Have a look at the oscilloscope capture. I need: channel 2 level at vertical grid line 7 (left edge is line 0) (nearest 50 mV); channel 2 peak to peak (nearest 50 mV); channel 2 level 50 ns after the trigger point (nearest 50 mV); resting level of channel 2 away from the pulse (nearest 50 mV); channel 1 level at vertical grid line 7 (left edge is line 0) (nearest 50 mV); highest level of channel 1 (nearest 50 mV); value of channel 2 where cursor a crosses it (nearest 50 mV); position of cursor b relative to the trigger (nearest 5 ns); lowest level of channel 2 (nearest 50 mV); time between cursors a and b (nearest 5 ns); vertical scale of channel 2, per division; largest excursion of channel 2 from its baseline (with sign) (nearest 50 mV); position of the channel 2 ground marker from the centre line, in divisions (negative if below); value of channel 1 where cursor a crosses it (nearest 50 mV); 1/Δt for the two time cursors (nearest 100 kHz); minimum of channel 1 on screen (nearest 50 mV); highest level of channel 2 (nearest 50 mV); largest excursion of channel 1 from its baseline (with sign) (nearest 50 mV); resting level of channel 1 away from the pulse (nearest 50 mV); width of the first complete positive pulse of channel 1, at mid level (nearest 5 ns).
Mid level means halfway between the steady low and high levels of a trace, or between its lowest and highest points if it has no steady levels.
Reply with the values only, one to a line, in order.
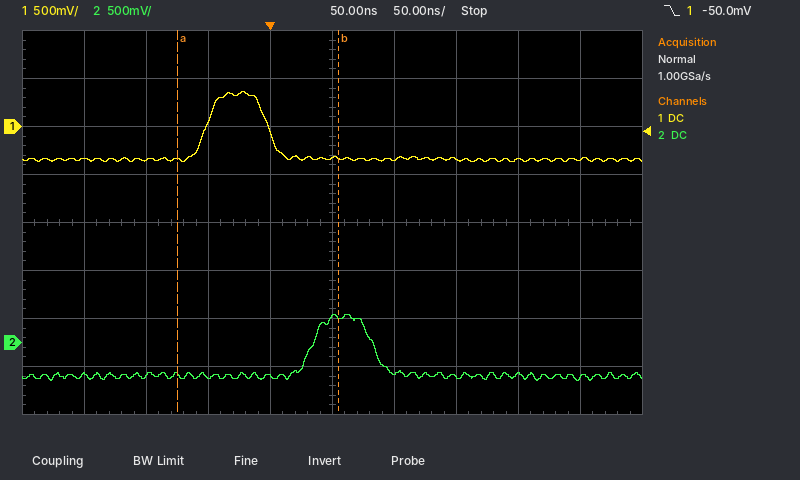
-350 mV
700 mV
250 mV
-350 mV
-350 mV
350 mV
-350 mV
+55 ns
-400 mV
130 ns
500 mV
+650 mV
-2.5 div
-350 mV
7.7 MHz
-350 mV
300 mV
+700 mV
-350 mV
50 ns
